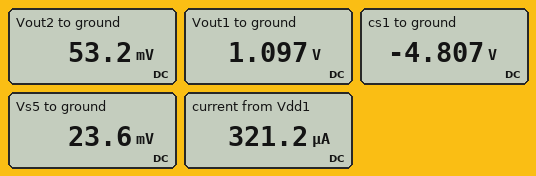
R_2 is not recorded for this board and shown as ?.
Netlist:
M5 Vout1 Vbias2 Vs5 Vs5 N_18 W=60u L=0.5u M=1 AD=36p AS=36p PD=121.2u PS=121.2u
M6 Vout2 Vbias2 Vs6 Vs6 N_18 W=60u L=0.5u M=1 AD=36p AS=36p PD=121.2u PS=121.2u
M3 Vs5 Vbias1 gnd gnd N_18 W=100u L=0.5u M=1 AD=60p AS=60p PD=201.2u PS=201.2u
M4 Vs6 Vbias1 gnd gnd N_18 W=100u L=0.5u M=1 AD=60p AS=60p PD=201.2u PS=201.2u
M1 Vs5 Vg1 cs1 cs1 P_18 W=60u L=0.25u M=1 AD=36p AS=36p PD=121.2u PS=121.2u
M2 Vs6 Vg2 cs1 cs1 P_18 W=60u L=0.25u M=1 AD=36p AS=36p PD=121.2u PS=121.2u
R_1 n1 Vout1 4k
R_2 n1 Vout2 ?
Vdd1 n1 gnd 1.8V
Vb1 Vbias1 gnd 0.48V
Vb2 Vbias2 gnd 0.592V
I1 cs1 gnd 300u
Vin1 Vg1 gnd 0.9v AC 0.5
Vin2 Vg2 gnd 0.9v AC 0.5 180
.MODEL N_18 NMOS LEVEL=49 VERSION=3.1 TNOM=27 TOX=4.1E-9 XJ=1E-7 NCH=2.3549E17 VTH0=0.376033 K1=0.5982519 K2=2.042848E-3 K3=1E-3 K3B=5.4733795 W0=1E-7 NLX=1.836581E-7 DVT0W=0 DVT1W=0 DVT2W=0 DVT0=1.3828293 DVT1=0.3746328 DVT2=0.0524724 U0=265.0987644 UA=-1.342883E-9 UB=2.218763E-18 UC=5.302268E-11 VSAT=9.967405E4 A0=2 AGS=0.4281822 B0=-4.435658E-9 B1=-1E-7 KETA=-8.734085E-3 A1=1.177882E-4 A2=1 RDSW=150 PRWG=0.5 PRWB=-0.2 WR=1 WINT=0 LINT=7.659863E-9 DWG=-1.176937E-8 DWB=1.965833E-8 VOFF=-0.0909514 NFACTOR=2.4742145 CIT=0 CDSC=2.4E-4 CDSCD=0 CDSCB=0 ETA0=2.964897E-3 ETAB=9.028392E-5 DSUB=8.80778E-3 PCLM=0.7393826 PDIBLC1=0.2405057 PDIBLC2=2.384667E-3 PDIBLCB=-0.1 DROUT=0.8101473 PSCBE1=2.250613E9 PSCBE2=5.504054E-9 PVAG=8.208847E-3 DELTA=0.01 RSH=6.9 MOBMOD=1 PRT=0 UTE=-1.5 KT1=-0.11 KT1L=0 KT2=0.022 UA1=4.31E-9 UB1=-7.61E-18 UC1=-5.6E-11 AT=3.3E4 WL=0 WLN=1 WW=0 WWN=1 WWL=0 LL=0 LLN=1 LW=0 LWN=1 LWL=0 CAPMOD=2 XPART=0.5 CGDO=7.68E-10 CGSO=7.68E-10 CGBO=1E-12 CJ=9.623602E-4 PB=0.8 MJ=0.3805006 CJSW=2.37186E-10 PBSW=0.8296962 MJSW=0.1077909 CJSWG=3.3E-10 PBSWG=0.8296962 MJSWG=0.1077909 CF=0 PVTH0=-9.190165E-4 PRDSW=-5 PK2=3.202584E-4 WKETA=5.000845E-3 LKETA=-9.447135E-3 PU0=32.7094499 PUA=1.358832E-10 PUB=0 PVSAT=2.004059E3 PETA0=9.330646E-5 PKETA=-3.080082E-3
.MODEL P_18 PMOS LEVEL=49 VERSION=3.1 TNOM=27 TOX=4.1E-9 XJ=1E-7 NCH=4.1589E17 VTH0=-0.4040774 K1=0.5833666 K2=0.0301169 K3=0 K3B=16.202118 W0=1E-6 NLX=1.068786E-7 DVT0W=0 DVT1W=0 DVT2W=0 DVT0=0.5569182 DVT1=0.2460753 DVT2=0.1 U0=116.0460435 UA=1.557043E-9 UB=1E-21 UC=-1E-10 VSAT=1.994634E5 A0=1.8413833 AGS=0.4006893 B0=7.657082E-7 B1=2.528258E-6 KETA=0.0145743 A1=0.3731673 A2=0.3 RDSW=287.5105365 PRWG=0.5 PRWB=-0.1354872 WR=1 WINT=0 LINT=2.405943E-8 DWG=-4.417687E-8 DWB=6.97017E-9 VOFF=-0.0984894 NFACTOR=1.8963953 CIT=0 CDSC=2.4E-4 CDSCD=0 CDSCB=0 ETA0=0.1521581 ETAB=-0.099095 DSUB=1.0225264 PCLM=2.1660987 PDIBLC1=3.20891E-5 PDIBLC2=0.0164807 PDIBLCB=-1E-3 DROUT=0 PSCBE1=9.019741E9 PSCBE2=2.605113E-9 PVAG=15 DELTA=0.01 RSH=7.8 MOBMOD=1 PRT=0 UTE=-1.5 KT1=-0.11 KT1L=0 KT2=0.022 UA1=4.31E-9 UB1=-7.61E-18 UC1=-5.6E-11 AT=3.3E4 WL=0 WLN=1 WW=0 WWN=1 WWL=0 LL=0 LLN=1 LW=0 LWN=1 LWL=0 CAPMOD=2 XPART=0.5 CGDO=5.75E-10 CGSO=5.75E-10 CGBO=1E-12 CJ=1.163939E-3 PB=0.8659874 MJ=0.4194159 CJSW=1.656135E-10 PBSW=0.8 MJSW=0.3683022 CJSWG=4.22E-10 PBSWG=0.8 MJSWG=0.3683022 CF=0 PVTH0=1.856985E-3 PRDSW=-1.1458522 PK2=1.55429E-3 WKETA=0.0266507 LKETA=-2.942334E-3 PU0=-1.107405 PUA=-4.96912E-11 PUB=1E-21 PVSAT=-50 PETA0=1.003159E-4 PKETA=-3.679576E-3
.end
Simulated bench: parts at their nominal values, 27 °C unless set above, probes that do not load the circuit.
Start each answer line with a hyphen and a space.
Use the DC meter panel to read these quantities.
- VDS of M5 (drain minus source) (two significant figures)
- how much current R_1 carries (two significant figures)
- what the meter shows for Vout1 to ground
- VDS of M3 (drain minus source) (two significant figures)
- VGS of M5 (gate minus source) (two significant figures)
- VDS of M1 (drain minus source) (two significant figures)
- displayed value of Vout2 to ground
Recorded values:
- 1.1 V
- 180 µA
- 1.097 V
- 24 mV
- 570 mV
- 4.8 V
- 53.2 mV
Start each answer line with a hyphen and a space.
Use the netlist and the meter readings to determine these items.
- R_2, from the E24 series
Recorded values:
- 12 kΩ
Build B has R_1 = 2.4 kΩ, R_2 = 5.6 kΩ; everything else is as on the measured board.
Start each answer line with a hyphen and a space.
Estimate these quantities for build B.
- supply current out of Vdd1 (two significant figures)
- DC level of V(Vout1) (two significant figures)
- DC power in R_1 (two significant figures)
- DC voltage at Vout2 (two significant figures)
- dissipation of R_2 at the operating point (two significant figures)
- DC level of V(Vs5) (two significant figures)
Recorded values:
- 350 µA
- 1.4 V
- 75 µW
- 830 mV
- 170 µW
- 26 mV
